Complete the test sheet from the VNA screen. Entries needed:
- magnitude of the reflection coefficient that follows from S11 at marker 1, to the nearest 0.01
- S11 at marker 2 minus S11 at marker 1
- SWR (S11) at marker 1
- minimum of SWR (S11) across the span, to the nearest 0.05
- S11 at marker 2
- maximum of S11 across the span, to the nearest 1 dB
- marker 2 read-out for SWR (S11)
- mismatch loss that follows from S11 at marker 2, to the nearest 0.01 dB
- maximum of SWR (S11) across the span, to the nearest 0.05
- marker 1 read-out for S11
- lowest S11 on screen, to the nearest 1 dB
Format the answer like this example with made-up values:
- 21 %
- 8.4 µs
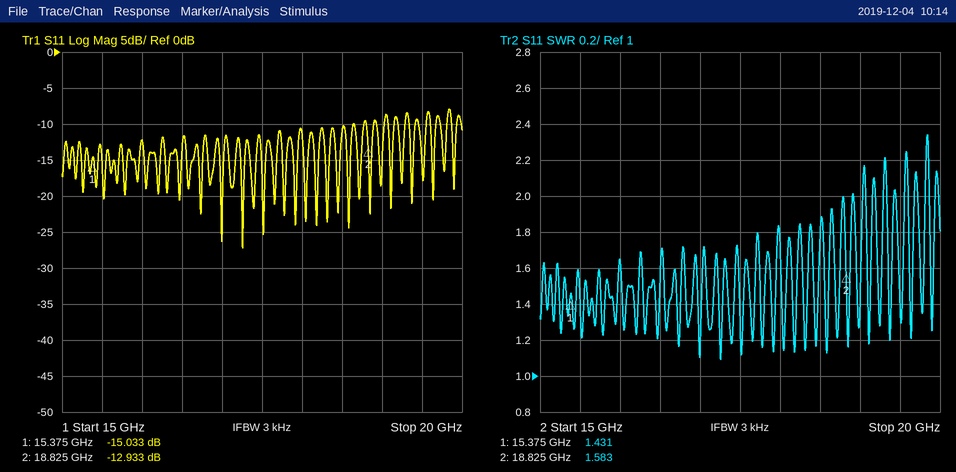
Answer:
- 0.18
- 2.100 dB
- 1.431
- 1.10
- -12.933 dB
- -8 dB
- 1.583
- 0.23 dB
- 2.35
- -15.033 dB
- -27 dB
